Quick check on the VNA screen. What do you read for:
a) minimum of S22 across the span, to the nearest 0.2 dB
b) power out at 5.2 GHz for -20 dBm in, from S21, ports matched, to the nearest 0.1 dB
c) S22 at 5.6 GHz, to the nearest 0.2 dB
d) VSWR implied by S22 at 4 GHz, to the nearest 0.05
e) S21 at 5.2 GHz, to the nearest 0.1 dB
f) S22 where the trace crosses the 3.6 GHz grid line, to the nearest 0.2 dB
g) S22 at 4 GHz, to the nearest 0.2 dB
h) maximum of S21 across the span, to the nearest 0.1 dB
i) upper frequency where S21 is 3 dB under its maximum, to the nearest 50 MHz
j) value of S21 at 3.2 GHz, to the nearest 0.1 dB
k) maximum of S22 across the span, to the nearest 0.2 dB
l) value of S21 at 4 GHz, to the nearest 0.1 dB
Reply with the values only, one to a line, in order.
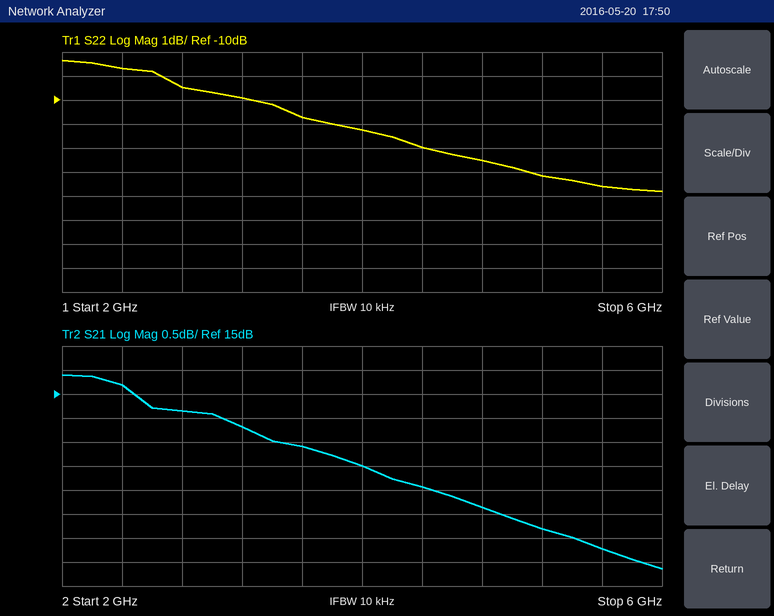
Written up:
-13.8 dB
-7.8 dBm
-13.6 dB
1.75
12.2 dB
-10.8 dB
-11.2 dB
15.4 dB
5.00 GHz
14.3 dB
-8.4 dB
13.5 dB
